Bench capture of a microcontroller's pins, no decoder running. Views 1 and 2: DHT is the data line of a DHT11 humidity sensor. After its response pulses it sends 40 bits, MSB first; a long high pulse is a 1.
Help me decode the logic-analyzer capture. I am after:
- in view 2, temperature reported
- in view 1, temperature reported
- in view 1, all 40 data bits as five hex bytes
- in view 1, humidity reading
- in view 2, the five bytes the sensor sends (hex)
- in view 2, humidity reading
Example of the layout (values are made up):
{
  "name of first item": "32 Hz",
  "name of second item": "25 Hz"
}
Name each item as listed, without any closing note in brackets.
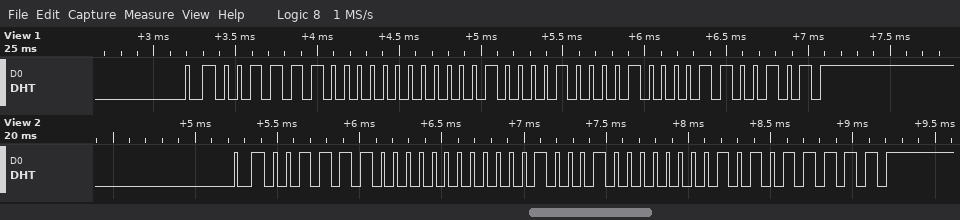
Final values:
{
  "in view 2, temperature reported": "34.1 °C",
  "in view 1, temperature reported": "33.8 °C",
  "in view 1, all 40 data bits as five hex bytes": "3C 00 21 08 65",
  "in view 1, humidity reading": "60 %",
  "in view 2, the five bytes the sensor sends": "3C 00 22 01 5F",
  "in view 2, humidity reading": "60 %"
}
